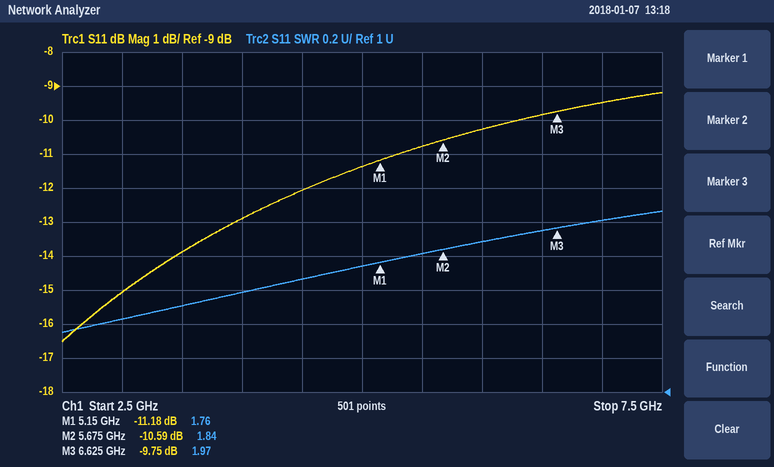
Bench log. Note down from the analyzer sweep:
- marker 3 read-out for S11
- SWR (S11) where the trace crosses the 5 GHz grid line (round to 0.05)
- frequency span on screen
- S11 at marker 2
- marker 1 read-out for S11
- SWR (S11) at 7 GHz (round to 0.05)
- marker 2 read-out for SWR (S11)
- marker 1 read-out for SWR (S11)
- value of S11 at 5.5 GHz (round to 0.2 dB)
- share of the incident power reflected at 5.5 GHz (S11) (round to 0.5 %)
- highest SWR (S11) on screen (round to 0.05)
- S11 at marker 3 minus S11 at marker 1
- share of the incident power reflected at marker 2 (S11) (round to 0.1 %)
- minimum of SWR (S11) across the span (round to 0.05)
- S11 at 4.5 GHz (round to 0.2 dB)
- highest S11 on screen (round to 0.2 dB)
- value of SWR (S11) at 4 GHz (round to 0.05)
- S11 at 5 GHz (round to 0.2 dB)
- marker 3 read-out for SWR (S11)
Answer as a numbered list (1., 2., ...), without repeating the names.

1. -9.75 dB
2. 1.75
3. 5 GHz
4. -10.59 dB
5. -11.18 dB
6. 2.00
7. 1.84
8. 1.76
9. -10.8 dB
10. 8.5 %
11. 2.05
12. 1.43 dB
13. 8.7 %
14. 1.35
15. -12.0 dB
16. -9.2 dB
17. 1.60
18. -11.4 dB
19. 1.97
